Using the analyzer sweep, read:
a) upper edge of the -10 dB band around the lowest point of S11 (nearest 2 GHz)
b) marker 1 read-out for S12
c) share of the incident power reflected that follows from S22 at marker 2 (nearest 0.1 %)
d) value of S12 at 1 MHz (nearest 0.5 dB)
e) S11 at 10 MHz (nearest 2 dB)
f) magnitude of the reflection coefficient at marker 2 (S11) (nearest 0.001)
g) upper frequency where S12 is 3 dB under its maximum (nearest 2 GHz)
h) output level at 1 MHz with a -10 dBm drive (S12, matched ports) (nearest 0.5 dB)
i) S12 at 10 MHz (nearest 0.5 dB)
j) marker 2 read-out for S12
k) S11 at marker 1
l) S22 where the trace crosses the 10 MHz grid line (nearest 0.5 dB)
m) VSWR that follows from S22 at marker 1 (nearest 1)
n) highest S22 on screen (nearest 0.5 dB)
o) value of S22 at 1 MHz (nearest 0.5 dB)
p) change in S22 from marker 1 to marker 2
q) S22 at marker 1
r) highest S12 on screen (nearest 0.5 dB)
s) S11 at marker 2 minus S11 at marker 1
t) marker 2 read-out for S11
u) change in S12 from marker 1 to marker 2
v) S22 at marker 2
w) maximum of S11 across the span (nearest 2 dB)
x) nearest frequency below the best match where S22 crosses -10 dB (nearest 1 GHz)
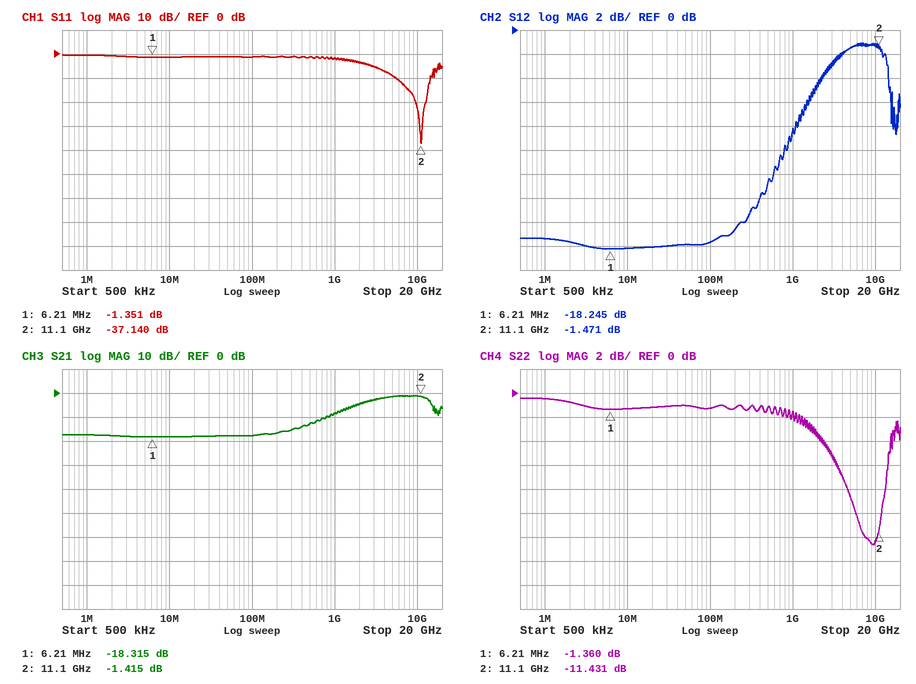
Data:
14 GHz
-18.245 dB
7.2 %
-17.5 dB
-2 dB
0.014
14 GHz
-27.5 dBm
-18.0 dB
-1.471 dB
-1.351 dB
-1.5 dB
13
-0.5 dB
-0.5 dB
-10.071 dB
-1.360 dB
-1.0 dB
-35.789 dB
-37.140 dB
16.774 dB
-11.431 dB
0 dB
6 GHz
